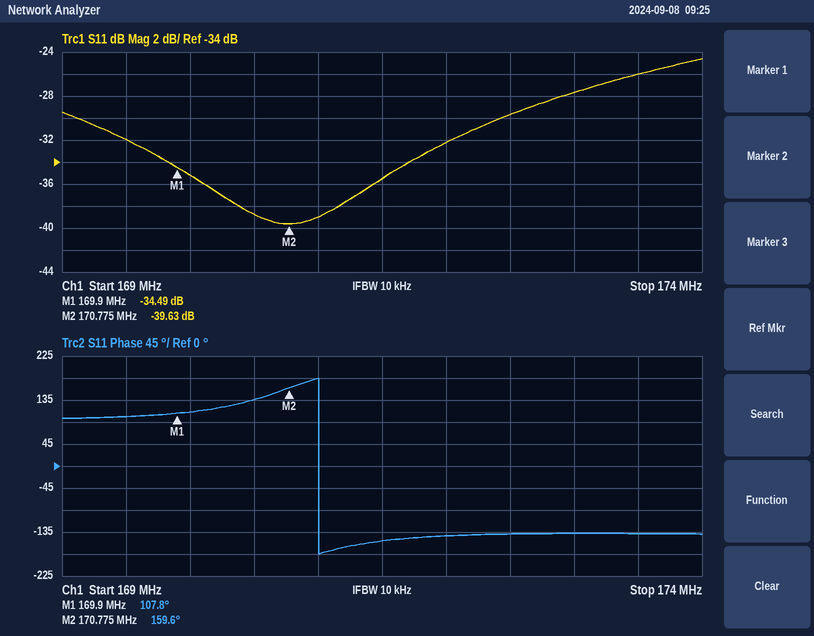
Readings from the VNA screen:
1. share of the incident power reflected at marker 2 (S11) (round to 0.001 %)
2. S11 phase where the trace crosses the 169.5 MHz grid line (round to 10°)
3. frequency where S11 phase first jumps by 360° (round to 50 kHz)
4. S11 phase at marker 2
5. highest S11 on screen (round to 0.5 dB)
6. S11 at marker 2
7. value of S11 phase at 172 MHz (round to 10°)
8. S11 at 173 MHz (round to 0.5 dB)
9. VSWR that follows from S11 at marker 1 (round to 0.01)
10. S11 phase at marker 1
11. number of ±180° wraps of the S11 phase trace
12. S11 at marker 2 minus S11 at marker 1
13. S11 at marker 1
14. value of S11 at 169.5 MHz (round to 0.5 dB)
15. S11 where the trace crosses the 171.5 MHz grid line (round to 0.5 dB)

0.011 %
100°
171.00 MHz
159.6°
-24.5 dB
-39.63 dB
-140°
-27.5 dB
1.04
107.8°
1
-5.14 dB
-34.49 dB
-32.0 dB
-35.5 dB
